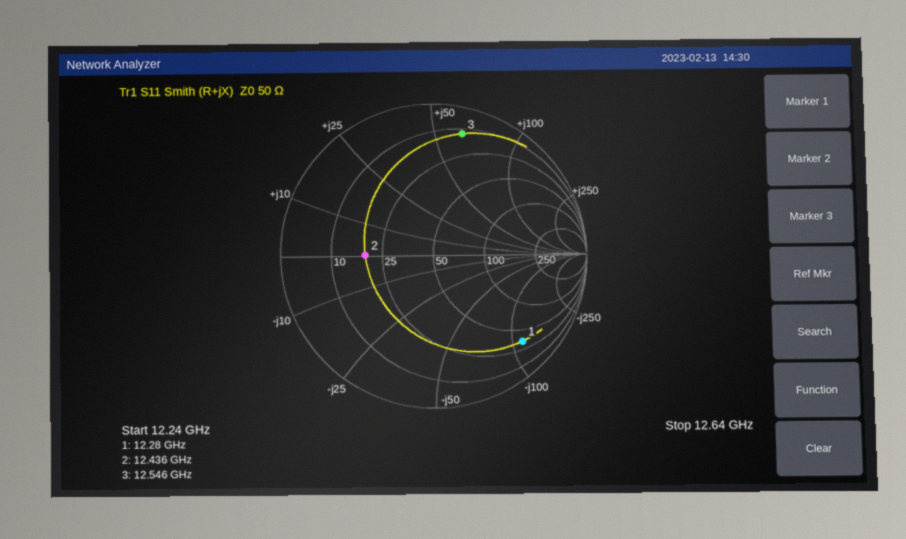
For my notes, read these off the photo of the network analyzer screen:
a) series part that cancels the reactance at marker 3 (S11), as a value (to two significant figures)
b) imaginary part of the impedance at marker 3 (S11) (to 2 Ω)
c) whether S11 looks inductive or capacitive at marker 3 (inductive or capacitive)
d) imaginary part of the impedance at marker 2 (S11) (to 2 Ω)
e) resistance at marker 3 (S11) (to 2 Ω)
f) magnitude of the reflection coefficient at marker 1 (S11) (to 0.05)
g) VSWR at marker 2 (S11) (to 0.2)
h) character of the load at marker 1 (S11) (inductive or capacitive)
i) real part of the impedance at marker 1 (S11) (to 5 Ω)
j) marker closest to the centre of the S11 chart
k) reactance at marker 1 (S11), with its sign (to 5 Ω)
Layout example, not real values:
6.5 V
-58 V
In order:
200 fF
+62 Ω
inductive
0 Ω
12 Ω
0.80
2.6
capacitive
35 Ω
marker 2
-110 Ω
